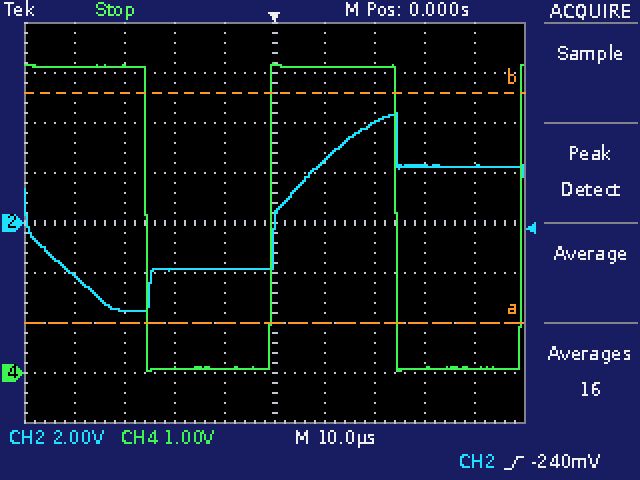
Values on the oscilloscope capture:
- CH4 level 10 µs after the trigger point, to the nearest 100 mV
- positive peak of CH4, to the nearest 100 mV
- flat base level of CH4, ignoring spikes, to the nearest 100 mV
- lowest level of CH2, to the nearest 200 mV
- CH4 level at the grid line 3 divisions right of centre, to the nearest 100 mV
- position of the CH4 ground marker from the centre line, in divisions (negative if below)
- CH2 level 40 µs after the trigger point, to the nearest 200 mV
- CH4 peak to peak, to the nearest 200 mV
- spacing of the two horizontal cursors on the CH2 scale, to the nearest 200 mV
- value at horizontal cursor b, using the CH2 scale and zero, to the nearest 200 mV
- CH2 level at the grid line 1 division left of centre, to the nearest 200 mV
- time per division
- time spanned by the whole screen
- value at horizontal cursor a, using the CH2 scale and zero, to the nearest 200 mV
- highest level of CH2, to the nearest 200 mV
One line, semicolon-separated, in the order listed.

6.1 V; 6.2 V; 100 mV; -3.6 V; 100 mV; -3.0 div; 2.2 V; 6.2 V; 9.2 V; 5.2 V; -1.8 V; 10 µs; 100 µs; -4.0 V; 4.4 V
